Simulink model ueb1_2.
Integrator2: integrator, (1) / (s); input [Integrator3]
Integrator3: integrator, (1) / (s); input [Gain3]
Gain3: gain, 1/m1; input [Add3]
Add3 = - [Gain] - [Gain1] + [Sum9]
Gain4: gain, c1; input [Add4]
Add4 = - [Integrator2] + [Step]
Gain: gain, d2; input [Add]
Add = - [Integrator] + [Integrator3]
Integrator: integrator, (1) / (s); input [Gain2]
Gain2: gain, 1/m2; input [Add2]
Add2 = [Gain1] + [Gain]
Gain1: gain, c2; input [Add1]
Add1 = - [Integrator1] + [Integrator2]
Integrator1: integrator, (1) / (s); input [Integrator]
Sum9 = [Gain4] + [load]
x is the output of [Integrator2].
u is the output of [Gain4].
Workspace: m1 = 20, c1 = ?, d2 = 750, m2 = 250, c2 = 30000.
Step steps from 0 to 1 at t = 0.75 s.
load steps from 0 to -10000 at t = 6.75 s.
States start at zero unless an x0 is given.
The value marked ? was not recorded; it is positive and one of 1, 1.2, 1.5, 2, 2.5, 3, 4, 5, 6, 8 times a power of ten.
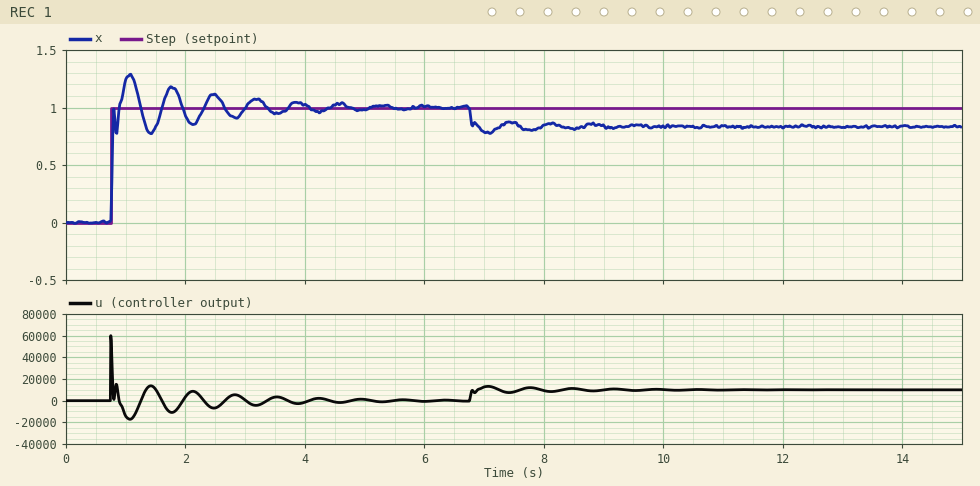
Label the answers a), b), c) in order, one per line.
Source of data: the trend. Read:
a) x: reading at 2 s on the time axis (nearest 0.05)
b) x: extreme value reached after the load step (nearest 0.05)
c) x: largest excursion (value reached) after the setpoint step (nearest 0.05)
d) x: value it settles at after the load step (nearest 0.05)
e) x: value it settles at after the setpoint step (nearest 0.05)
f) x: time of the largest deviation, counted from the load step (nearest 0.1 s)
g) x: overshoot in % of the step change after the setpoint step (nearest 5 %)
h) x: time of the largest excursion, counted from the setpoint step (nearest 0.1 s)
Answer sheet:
a) 0.95
b) 0.80
c) 1.30
d) 0.85
e) 1.00
f) 0.3 s
g) 30 %
h) 0.3 s
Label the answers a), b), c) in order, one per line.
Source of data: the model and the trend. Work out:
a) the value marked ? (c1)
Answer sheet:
a) 60000
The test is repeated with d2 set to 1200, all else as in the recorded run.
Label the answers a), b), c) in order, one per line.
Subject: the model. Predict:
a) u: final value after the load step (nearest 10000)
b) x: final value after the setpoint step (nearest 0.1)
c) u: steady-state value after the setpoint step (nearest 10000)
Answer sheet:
a) 10000
b) 1.0
c) 0
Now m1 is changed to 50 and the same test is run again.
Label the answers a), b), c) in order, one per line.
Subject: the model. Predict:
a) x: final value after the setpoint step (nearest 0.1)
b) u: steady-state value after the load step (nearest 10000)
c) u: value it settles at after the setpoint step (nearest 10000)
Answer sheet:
a) 1.0
b) 10000
c) 0
